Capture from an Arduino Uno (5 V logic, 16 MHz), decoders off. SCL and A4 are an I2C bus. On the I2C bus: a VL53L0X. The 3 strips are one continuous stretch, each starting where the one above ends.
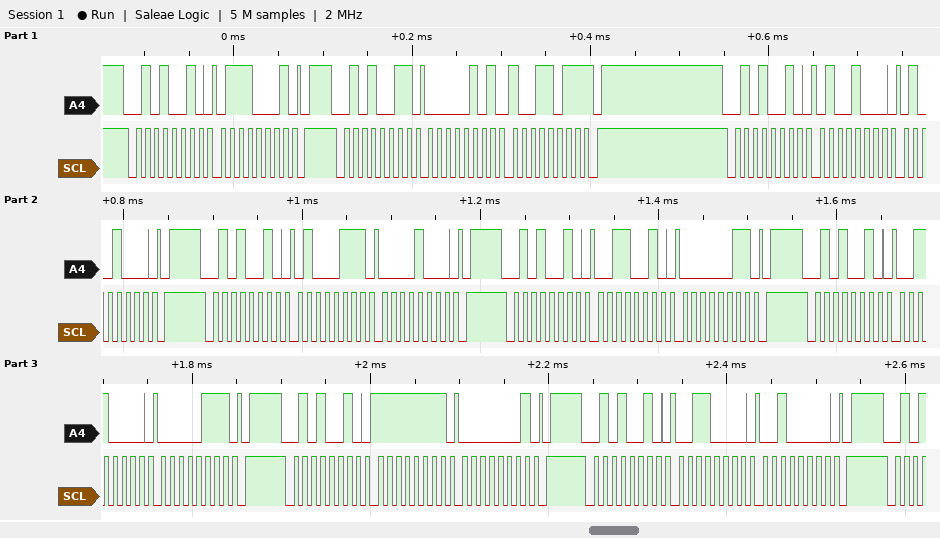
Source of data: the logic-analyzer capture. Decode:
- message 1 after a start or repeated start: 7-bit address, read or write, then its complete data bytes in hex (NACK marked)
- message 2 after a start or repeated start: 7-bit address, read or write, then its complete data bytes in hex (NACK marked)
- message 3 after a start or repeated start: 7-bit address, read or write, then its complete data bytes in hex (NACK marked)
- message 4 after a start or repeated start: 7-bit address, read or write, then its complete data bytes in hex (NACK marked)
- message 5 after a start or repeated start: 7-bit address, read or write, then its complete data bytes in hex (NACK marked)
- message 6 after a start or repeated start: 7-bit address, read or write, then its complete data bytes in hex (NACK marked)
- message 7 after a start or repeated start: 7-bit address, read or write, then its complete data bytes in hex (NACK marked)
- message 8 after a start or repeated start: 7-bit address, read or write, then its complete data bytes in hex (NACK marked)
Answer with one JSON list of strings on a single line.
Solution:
["0x29 write: 71", "0x29 read: 05 9B NACK", "0x29 write: 48 48", "0x29 write: 47 08", "0x29 write: 32 03", "0x29 write: 30 07", "0x29 write: FF 01", "0x29 write: 30 20"]
